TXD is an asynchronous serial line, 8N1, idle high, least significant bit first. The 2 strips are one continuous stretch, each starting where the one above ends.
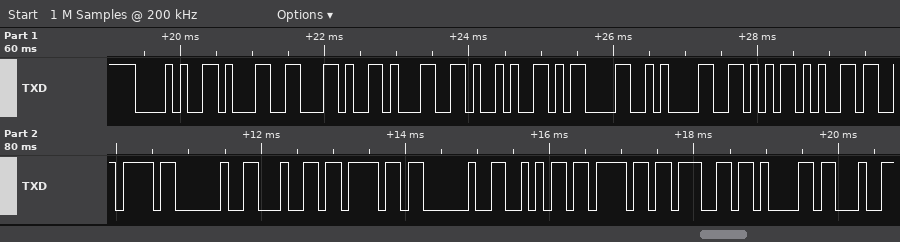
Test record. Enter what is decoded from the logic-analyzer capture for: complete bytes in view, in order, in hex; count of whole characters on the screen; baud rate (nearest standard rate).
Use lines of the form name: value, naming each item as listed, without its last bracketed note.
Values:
complete bytes in view, in order, in hex: 28 31 2C 31 29 0D 0A 56 65 7A 20 64 6F 20 6A 6F 67 61
count of whole characters on the screen: 18
baud rate: 9600 baud
